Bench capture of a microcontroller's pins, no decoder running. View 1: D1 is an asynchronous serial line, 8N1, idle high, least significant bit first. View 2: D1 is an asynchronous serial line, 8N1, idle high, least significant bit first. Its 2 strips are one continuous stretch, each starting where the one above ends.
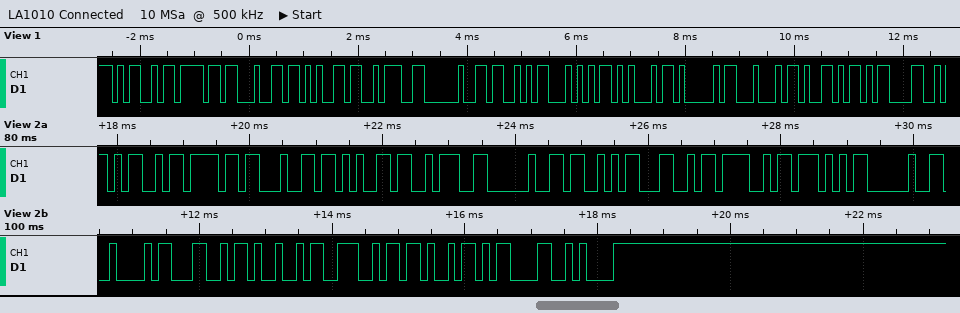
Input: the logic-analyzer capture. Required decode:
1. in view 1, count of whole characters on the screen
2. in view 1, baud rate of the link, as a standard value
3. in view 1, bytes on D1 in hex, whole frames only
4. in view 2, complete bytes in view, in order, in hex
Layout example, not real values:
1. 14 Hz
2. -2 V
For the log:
1. 13
2. 9600 baud
3. 4D 6F 64 65 3A 20 53 54 45 41 44 59 0D
4. 4D 6F 64 65 3A 20 53 4C 4F 57 20 42 4C 49 4E 4B 0D 0A
